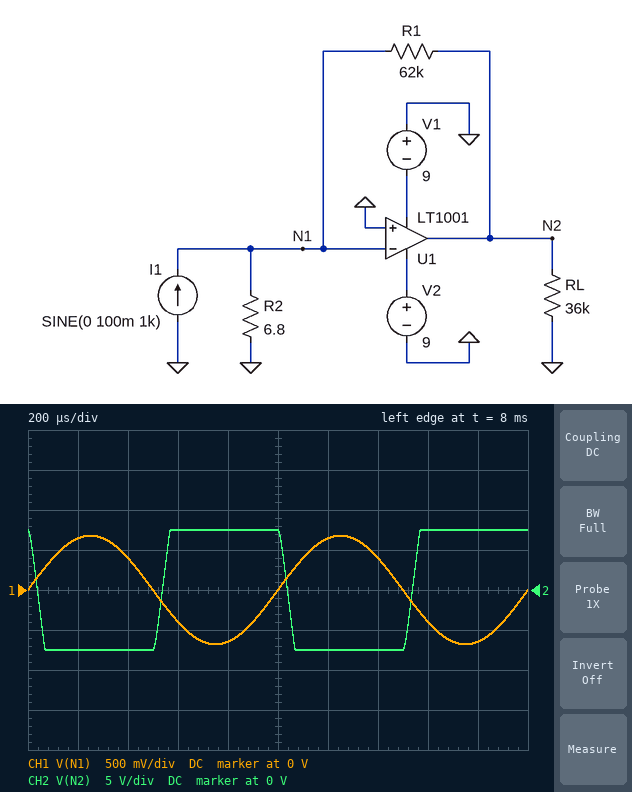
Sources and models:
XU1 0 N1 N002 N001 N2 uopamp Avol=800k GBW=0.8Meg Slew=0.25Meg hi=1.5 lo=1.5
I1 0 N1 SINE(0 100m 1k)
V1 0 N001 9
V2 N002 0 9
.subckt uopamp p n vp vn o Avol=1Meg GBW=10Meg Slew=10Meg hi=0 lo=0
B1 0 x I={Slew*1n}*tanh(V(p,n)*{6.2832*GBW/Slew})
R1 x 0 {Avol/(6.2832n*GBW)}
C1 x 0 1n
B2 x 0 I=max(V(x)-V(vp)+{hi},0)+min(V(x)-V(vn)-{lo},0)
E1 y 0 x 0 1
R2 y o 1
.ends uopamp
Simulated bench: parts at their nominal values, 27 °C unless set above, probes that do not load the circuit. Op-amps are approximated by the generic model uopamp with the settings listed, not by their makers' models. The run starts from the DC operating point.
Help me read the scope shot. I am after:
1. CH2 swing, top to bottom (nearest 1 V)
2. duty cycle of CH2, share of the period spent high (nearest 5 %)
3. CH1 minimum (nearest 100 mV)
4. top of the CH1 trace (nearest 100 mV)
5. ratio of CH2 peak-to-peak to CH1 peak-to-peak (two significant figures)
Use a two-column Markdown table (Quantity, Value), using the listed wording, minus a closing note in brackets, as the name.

| Quantity | Value |
|---|---|
| CH2 swing, top to bottom | 15 V |
| duty cycle of CH2, share of the period spent high | 50 % |
| CH1 minimum | -700 mV |
| top of the CH1 trace | 700 mV |
| ratio of CH2 peak-to-peak to CH1 peak-to-peak | 11 |
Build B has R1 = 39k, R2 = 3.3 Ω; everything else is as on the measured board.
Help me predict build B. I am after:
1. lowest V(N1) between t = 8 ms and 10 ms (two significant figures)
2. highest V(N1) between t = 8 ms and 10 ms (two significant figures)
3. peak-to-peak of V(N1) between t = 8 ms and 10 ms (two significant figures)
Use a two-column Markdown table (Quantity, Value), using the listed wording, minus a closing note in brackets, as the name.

| Quantity | Value |
|---|---|
| lowest V(N1) between t = 8 ms and 10 ms | -330 mV |
| highest V(N1) between t = 8 ms and 10 ms | 330 mV |
| peak-to-peak of V(N1) between t = 8 ms and 10 ms | 660 mV |
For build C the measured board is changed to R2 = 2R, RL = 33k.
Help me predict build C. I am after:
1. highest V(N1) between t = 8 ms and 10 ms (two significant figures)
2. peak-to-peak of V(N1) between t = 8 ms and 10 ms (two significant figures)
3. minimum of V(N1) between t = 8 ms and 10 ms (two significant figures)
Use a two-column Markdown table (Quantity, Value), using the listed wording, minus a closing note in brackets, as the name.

| Quantity | Value |
|---|---|
| highest V(N1) between t = 8 ms and 10 ms | 200 mV |
| peak-to-peak of V(N1) between t = 8 ms and 10 ms | 400 mV |
| minimum of V(N1) between t = 8 ms and 10 ms | -200 mV |
